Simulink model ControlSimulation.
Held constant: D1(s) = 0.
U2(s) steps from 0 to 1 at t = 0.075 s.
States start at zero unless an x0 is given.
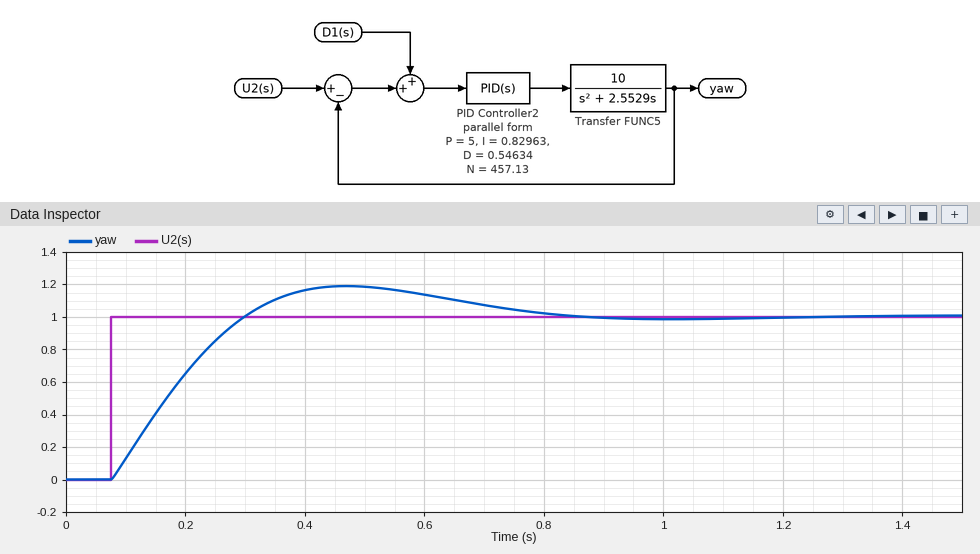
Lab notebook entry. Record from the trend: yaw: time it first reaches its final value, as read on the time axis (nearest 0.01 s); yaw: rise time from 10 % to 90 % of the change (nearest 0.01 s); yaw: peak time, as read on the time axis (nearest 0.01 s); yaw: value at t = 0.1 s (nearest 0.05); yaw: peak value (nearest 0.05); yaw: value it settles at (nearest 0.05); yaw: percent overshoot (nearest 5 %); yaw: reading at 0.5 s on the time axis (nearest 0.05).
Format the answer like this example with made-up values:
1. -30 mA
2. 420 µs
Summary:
1. 0.30 s
2. 0.17 s
3. 0.47 s
4. 0.15
5. 1.20
6. 1.00
7. 20 %
8. 1.20
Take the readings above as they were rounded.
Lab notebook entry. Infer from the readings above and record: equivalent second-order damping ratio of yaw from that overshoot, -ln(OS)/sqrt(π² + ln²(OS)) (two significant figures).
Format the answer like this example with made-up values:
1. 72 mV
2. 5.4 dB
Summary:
1. 0.46
